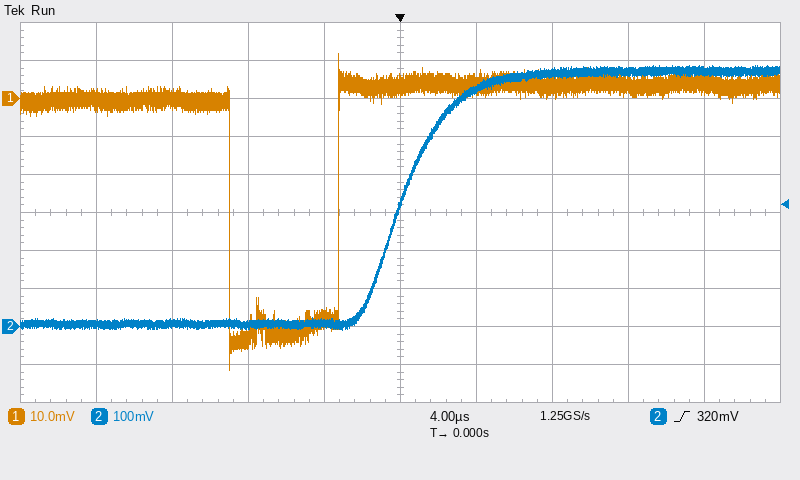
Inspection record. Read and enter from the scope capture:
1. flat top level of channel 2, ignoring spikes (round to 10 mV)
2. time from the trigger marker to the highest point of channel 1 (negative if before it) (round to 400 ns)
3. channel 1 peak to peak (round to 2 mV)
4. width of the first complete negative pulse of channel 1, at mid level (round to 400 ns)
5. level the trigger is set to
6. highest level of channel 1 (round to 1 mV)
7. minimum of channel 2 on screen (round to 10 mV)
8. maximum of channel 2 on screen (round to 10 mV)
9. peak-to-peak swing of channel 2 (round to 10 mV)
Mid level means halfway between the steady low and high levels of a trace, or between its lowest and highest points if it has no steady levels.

670 mV
-3.2 µs
84 mV
5.6 µs
320 mV
12 mV
-10 mV
690 mV
700 mV
